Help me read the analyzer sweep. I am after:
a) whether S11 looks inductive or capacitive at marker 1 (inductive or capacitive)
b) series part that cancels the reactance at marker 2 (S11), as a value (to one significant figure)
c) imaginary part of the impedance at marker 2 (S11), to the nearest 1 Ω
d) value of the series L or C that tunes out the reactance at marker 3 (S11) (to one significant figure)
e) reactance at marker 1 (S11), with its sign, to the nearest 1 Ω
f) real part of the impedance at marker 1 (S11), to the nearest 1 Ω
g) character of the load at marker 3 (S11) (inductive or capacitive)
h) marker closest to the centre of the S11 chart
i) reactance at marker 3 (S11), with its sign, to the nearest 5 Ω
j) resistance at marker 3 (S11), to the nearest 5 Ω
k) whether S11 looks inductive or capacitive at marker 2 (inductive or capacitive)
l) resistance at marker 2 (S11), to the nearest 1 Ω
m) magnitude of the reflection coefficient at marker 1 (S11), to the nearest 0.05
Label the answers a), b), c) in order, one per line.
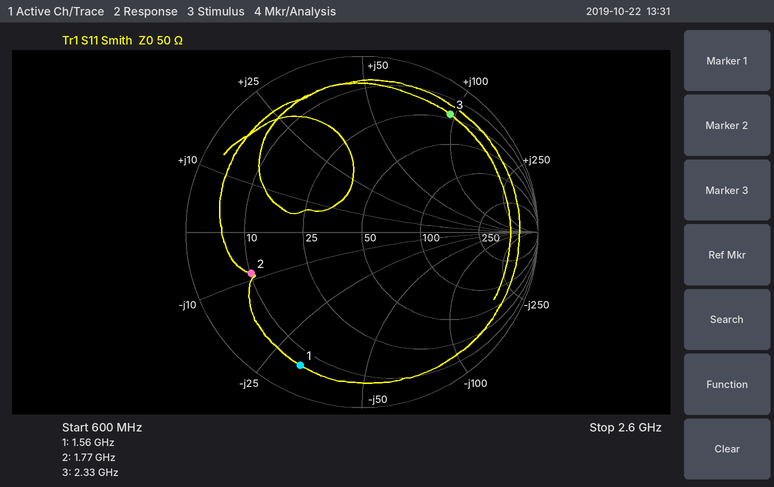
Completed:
a) capacitive
b) 800 pH
c) -9 Ω
d) 700 fF
e) -32 Ω
f) 6 Ω
g) inductive
h) marker 2
i) +95 Ω
j) 20 Ω
k) capacitive
l) 10 Ω
m) 0.85
